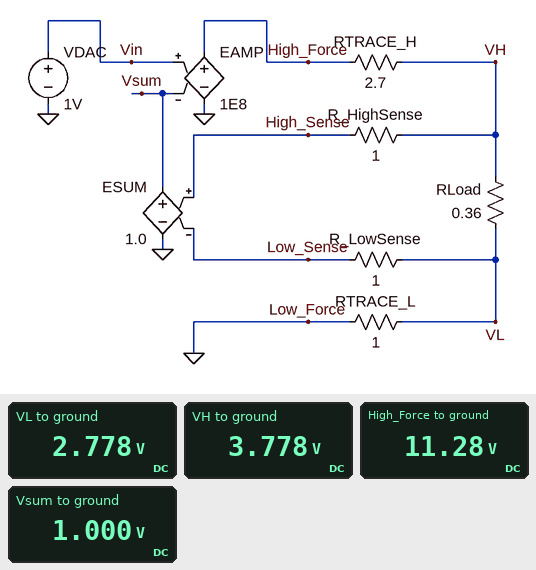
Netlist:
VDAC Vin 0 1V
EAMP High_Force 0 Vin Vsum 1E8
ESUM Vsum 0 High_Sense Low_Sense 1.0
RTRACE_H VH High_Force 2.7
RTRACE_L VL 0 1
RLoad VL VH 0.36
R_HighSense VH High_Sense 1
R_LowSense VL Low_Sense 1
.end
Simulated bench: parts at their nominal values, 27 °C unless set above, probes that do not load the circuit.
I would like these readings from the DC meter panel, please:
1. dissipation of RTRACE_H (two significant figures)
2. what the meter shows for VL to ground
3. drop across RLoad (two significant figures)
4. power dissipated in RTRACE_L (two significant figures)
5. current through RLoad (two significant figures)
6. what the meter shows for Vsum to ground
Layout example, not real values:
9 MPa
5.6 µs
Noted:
21 W
2.778 V
1.0 V
7.7 W
2.8 A
1.000 V
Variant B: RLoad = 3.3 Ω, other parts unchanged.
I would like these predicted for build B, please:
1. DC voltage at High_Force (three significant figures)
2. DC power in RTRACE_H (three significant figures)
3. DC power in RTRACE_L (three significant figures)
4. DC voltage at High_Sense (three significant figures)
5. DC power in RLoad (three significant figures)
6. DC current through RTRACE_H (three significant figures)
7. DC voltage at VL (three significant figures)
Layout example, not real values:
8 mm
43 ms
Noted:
2.12 V
248 mW
91.8 mW
1.30 V
303 mW
303 mA
303 mV
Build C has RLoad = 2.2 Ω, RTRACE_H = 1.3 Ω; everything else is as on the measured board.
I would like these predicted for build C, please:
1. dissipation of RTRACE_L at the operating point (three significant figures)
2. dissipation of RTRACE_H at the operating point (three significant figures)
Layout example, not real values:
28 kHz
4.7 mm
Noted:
207 mW
269 mW
